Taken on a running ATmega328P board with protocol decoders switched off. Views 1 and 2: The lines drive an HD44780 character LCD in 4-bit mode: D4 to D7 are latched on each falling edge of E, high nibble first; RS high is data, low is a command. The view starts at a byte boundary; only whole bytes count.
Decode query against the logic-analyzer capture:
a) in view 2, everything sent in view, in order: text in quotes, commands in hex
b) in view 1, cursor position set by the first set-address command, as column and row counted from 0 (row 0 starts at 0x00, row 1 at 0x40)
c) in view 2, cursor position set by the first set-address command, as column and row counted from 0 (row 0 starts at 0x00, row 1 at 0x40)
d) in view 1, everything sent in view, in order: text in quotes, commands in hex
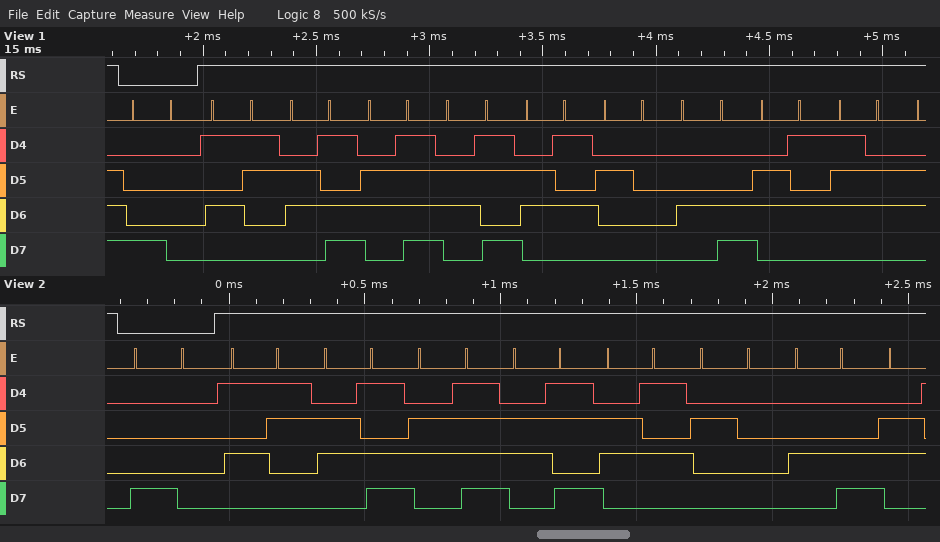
0x80 "Smoke L"
column 0, row 0
column 0, row 0
0x80 "Smoke Lev"
